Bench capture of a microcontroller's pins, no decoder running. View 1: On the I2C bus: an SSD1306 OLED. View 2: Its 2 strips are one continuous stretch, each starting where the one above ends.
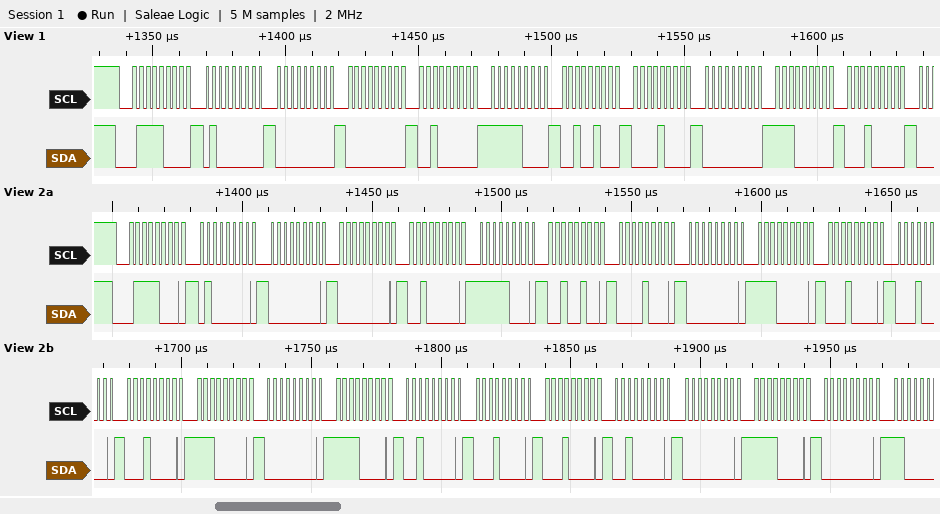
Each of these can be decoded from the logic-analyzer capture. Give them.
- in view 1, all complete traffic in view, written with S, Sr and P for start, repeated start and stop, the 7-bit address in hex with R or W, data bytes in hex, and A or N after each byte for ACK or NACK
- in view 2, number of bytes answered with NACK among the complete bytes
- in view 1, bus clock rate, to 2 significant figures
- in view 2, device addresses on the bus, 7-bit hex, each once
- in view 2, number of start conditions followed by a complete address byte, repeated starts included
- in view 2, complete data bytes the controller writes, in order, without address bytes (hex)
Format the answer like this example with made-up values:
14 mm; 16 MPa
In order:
S 3CW A 40 A 00 A 00 A 20 A F8 A 24 A 08 A 00 A E0 A 10 A; 0; 400 kHz; 0x3C; 1; 40 00 00 20 F8 24 08 00 E0 10 10 10 E0 00 F0 20 10 10 20 00 F0 00
